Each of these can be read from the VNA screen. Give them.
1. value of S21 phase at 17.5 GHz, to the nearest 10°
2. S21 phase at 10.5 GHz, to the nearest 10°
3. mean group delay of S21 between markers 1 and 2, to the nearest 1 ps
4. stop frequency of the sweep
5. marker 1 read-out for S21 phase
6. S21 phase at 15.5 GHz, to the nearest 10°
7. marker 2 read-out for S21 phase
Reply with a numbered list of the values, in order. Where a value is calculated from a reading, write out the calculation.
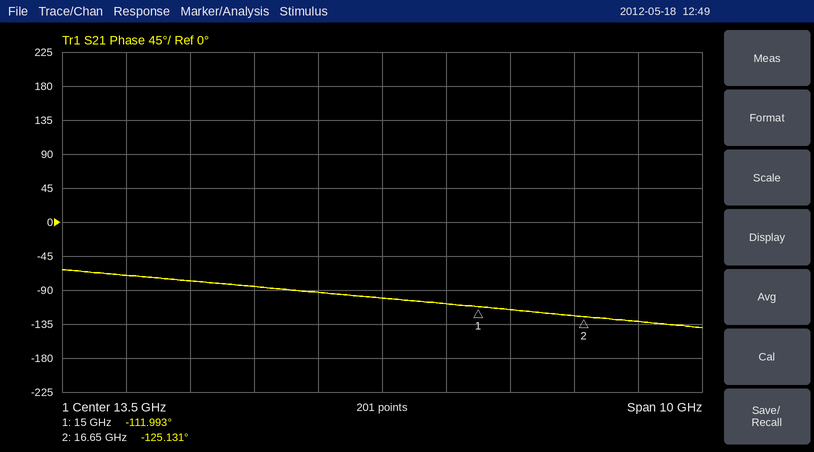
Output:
1. -130°
2. -80°
3. −(-125.131° − (-111.993°))/(360° × 1.65 GHz) ≈ 22 ps
4. 18.5 GHz
5. -111.993°
6. -120°
7. -125.131°
